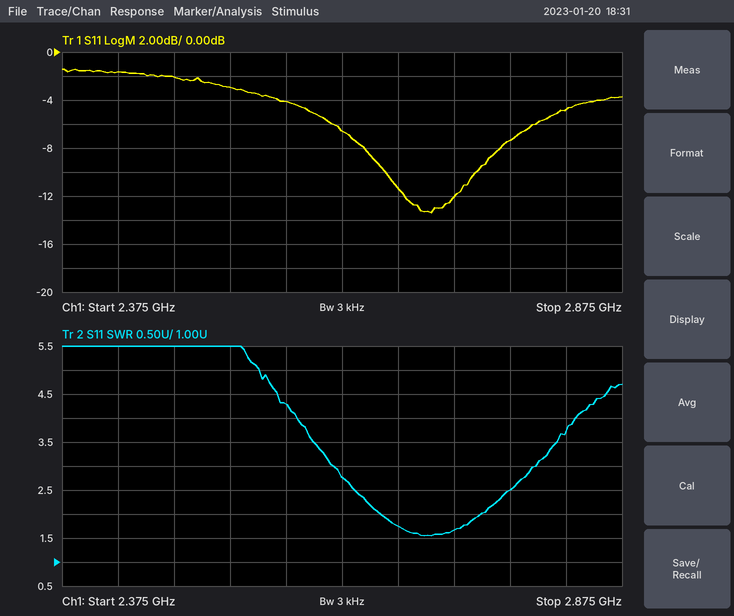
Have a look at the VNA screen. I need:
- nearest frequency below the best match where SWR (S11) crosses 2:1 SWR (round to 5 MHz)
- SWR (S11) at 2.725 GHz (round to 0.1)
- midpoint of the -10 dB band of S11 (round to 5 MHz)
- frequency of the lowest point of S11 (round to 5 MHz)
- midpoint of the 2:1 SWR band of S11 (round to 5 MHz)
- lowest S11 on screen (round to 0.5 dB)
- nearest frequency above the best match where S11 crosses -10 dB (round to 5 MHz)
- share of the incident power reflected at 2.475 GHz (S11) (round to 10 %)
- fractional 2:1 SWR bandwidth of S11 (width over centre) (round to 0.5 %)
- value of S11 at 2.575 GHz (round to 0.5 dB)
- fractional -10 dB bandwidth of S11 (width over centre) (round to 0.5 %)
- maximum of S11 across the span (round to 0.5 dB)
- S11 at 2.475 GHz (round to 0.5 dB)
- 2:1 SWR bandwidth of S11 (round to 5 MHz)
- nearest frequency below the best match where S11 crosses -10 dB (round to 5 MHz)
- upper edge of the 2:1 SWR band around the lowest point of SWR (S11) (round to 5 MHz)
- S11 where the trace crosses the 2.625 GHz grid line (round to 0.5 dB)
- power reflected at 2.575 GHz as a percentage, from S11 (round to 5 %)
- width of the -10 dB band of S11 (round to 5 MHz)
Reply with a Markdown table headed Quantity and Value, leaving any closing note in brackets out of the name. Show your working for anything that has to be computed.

| Quantity | Value |
|---|---|
| nearest frequency below the best match where SWR (S11) crosses 2:1 SWR | 2.660 GHz |
| SWR (S11) at 2.725 GHz | 1.7 |
| midpoint of the -10 dB band of S11 | 2.705 GHz |
| frequency of the lowest point of S11 | 2.705 GHz |
| midpoint of the 2:1 SWR band of S11 | 2.705 GHz |
| lowest S11 on screen | -13.5 dB |
| nearest frequency above the best match where S11 crosses -10 dB | 2.745 GHz |
| share of the incident power reflected at 2.475 GHz (S11) | 10^(-2/10) ≈ 63.1 %, so 60 % to the nearest 10 % |
| fractional 2:1 SWR bandwidth of S11 (width over centre) | 90 MHz / 2.705 GHz ≈ 3.33 %, so 3.5 % to the nearest 0.5 % |
| value of S11 at 2.575 GHz | -4.0 dB |
| fractional -10 dB bandwidth of S11 (width over centre) | 80 MHz / 2.705 GHz ≈ 3.0 % |
| maximum of S11 across the span | -1.5 dB |
| S11 at 2.475 GHz | -2.0 dB |
| 2:1 SWR bandwidth of S11 | 2.750 GHz − 2.660 GHz = 90 MHz |
| nearest frequency below the best match where S11 crosses -10 dB | 2.665 GHz |
| upper edge of the 2:1 SWR band around the lowest point of SWR (S11) | 2.750 GHz |
| S11 where the trace crosses the 2.625 GHz grid line | -6.5 dB |
| power reflected at 2.575 GHz as a percentage, from S11 | 10^(-4/10) ≈ 40 % |
| width of the -10 dB band of S11 | 2.745 GHz − 2.665 GHz = 80 MHz |
